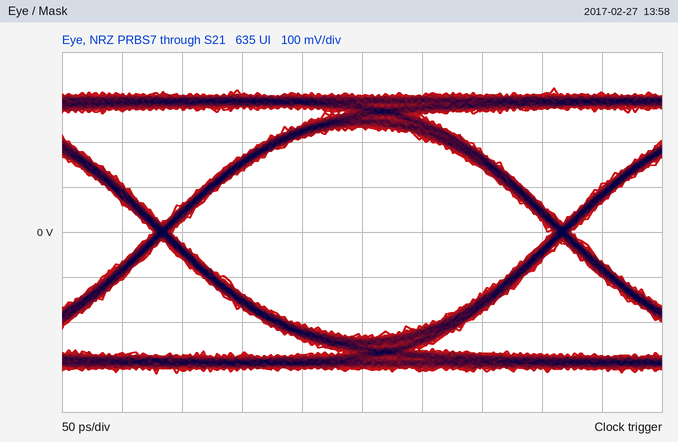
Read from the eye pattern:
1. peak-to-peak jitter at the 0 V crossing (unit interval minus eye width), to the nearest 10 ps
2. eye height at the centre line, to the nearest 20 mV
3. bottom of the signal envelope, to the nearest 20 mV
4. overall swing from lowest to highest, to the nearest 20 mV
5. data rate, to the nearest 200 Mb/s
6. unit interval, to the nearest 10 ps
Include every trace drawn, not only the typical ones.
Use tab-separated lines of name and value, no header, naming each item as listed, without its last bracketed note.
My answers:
peak-to-peak jitter at the 0 V crossing (unit interval minus eye width), to the nearest 10 ps	20 ps
eye height at the centre line, to the nearest 20 mV	460 mV
bottom of the signal envelope, to the nearest 20 mV	-320 mV
overall swing from lowest to highest, to the nearest 20 mV	640 mV
data rate, to the nearest 200 Mb/s	3.0 Gb/s
unit interval, to the nearest 10 ps	330 ps
